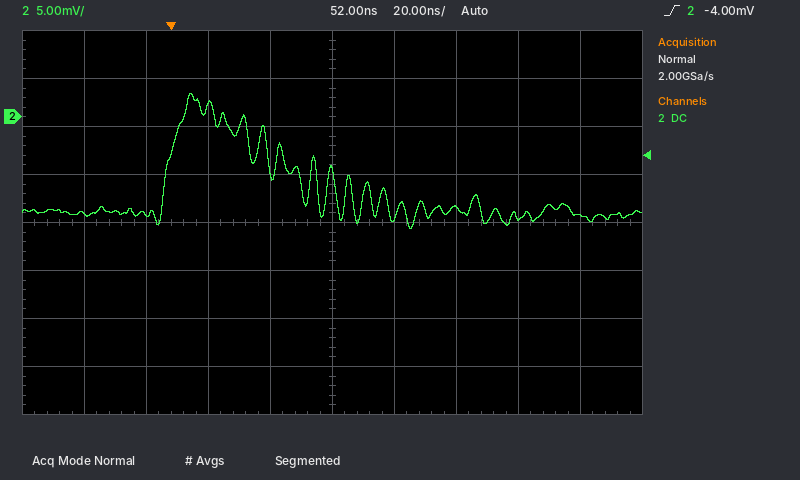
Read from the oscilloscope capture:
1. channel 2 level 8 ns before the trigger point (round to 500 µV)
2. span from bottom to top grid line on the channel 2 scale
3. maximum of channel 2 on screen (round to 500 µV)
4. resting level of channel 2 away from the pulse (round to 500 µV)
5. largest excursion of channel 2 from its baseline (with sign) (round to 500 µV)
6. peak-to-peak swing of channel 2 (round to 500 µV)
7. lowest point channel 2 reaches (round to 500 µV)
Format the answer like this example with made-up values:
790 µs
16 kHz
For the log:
-10.0 mV
40 mV
2.5 mV
-10.0 mV
+12.5 mV
14.0 mV
-11.5 mV
